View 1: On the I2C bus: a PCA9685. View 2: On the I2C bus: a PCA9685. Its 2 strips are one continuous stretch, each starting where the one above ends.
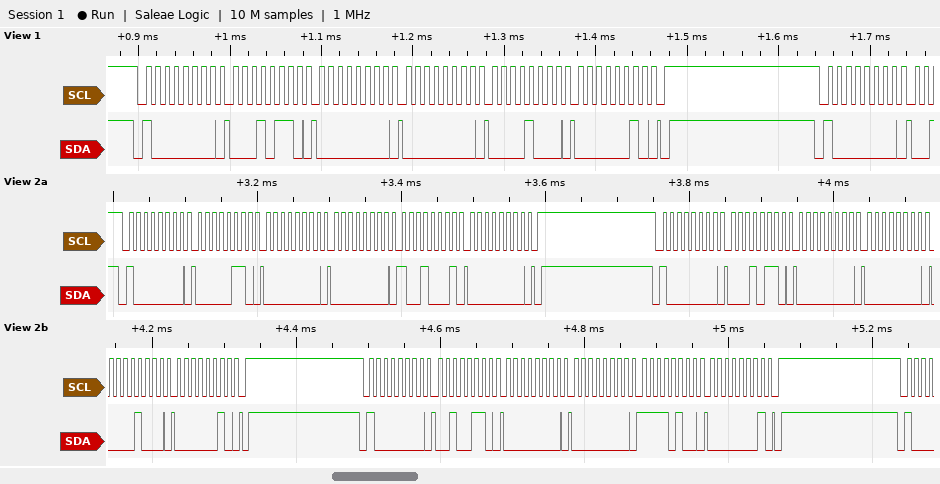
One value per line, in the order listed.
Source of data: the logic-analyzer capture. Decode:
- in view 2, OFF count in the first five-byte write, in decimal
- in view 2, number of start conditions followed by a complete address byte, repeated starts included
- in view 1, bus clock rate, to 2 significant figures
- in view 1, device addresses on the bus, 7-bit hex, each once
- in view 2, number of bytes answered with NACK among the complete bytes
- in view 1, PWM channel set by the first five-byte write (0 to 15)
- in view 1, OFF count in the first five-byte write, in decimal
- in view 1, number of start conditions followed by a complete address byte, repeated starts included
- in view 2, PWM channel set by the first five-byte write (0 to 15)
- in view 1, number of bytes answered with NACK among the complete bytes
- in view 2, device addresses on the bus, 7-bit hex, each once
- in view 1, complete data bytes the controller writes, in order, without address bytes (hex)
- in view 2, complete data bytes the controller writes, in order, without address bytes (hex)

145
3
100 kHz
0x40
0
4
520
2
0
0
0x40
16 00 00 08 02
06 00 00 91 00 16 00 00 08 02 26 00 00 F4 01
